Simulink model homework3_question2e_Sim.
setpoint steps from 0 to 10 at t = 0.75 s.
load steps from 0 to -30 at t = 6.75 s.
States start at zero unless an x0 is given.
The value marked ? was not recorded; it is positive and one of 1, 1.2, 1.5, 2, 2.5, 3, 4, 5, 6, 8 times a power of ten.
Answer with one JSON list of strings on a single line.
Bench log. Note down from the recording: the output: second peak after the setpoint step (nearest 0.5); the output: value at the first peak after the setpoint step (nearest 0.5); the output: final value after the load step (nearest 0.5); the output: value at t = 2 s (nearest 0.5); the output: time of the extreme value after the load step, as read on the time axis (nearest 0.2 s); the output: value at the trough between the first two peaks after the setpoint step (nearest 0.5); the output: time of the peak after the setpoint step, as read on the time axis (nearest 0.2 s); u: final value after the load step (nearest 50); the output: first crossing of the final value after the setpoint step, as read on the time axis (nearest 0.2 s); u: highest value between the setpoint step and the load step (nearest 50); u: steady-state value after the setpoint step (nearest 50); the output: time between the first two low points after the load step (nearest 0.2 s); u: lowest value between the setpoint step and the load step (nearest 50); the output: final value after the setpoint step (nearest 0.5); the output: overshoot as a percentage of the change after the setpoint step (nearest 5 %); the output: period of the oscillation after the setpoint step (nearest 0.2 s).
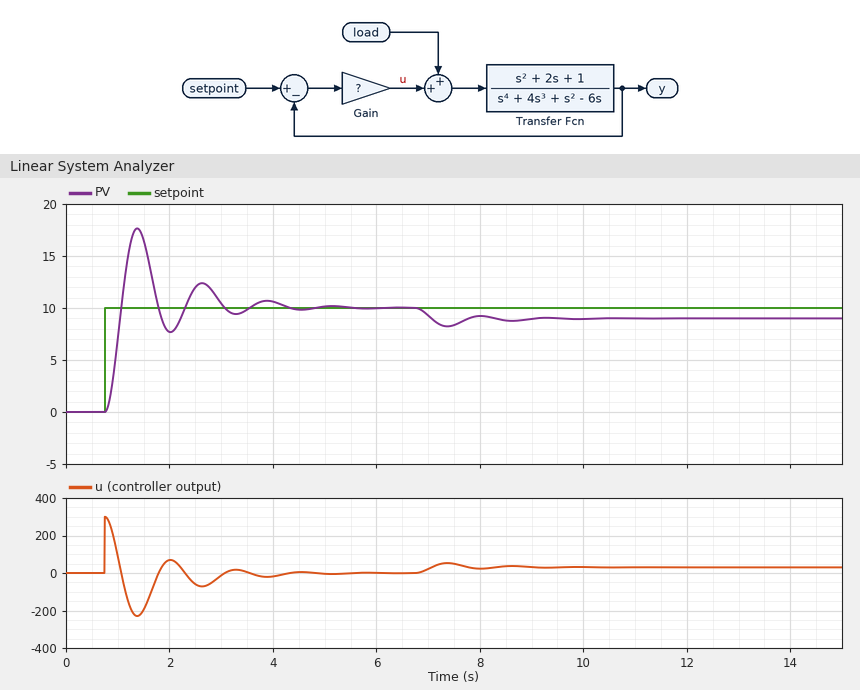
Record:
["12.5", "17.5", "9.0", "7.5", "7.4 s", "7.5", "1.4 s", "50", "1.0 s", "300", "0", "1.2 s", "-250", "10.0", "75 %", "1.2 s"]
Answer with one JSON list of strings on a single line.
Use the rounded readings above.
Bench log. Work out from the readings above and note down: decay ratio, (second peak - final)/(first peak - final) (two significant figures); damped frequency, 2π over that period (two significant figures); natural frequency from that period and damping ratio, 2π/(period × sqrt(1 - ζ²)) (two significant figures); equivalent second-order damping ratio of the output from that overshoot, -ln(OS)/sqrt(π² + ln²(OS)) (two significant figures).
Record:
["0.33", "5.2 rad/s", "5.3 rad/s", "0.091"]
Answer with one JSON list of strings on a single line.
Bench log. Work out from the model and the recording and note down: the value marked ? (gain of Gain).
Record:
["30"]
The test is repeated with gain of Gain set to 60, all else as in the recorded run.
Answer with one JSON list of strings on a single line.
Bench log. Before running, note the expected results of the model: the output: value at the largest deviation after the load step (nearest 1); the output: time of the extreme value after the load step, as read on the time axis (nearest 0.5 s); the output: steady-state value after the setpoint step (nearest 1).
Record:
["9", "7.0 s", "10"]
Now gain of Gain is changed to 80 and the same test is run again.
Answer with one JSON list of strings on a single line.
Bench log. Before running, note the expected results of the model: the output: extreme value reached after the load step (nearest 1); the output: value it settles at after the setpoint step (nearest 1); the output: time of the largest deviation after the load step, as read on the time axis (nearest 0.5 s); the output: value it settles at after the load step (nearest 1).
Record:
["9", "10", "7.0 s", "10"]
